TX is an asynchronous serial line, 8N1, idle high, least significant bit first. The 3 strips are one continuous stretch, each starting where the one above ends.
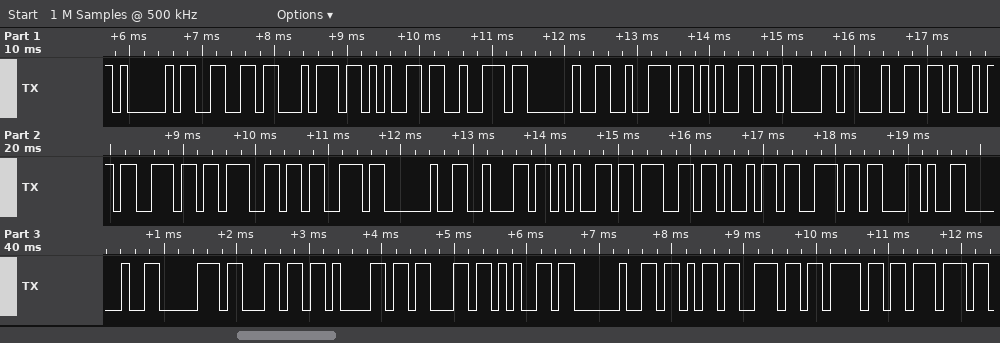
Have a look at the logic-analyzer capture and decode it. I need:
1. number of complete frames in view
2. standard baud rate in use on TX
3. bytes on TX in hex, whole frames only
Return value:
32
9600 baud
0x41 0x66 0x74 0x65 0x72 0x20 0x72 0x65 0x61 0x64 0x69 0x6E 0x67 0x73 0x20 0x62 0x65 0x67 0x69 0x6E 0x2C 0x20 0x70 0x6C 0x61 0x63 0x65 0x20 0x6B 0x6E 0x6F 0x77
